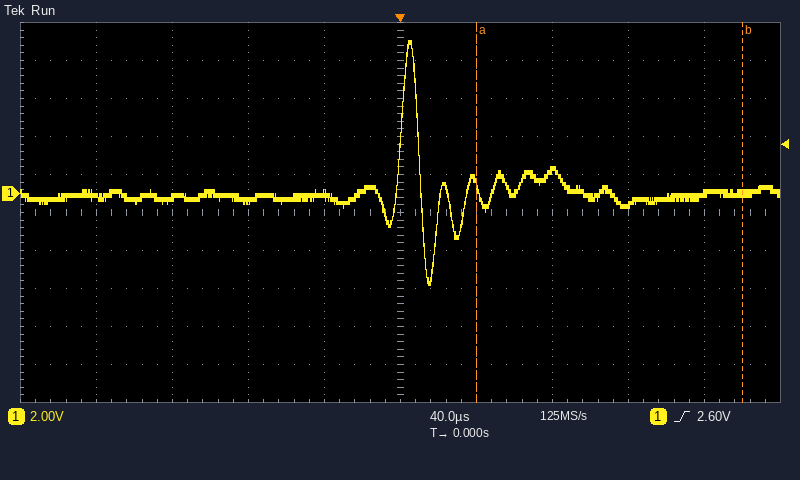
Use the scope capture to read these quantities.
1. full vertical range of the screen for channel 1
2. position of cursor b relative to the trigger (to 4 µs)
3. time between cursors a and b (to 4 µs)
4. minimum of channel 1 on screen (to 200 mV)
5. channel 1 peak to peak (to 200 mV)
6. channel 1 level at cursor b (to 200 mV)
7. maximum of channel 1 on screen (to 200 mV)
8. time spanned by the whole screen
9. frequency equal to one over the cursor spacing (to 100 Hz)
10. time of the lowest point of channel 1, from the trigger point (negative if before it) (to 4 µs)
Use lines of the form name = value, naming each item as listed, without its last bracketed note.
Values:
full vertical range of the screen for channel 1 = 20 V
position of cursor b relative to the trigger = +180 µs
time between cursors a and b = 140 µs
minimum of channel 1 on screen = -4.8 V
channel 1 peak to peak = 12.8 V
channel 1 level at cursor b = 0.0 V
maximum of channel 1 on screen = 8.0 V
time spanned by the whole screen = 400 µs
frequency equal to one over the cursor spacing = 7.1 kHz
time of the lowest point of channel 1, from the trigger point (negative if before it) = +16 µs
